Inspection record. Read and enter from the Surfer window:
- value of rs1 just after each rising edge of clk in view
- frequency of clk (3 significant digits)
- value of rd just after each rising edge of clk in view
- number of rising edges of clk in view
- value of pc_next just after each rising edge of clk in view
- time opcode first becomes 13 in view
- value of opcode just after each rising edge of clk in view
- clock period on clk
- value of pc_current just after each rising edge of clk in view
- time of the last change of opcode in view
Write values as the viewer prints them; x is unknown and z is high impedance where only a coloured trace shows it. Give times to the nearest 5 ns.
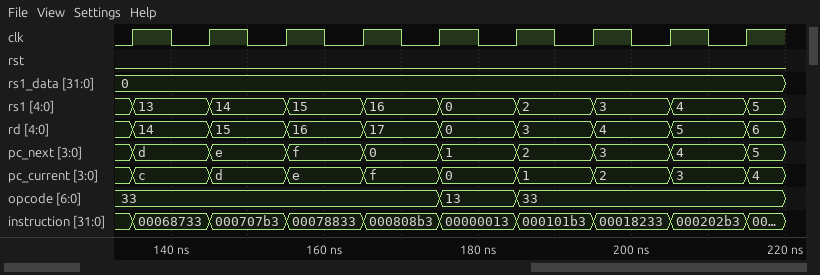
13, 14, 15, 16, 0, 2, 3, 4, 5
100 MHz
14, 15, 16, 17, 0, 3, 4, 5, 6
9
d, e, f, 0, 1, 2, 3, 4, 5
175 ns
33, 33, 33, 33, 13, 33, 33, 33, 33
10 ns
c, d, e, f, 0, 1, 2, 3, 4
185 ns
